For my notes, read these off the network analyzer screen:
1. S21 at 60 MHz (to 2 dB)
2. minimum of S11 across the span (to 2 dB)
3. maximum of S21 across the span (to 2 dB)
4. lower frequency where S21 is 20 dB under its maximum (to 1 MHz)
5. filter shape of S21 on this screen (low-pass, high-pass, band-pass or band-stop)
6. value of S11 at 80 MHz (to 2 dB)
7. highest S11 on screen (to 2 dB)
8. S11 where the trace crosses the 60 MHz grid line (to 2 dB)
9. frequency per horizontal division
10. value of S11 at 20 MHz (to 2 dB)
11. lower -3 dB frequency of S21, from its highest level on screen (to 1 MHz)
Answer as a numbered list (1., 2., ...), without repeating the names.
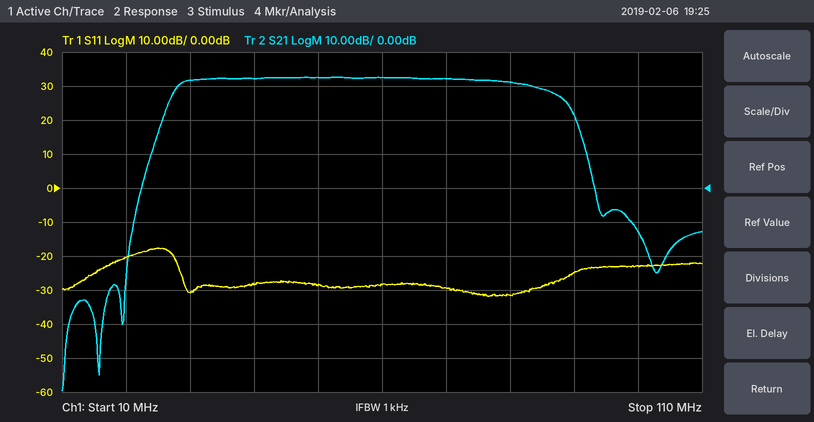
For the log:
1. 32 dB
2. -32 dB
3. 32 dB
4. 24 MHz
5. band-pass
6. -32 dB
7. -18 dB
8. -28 dB
9. 10 MHz
10. -20 dB
11. 28 MHz
